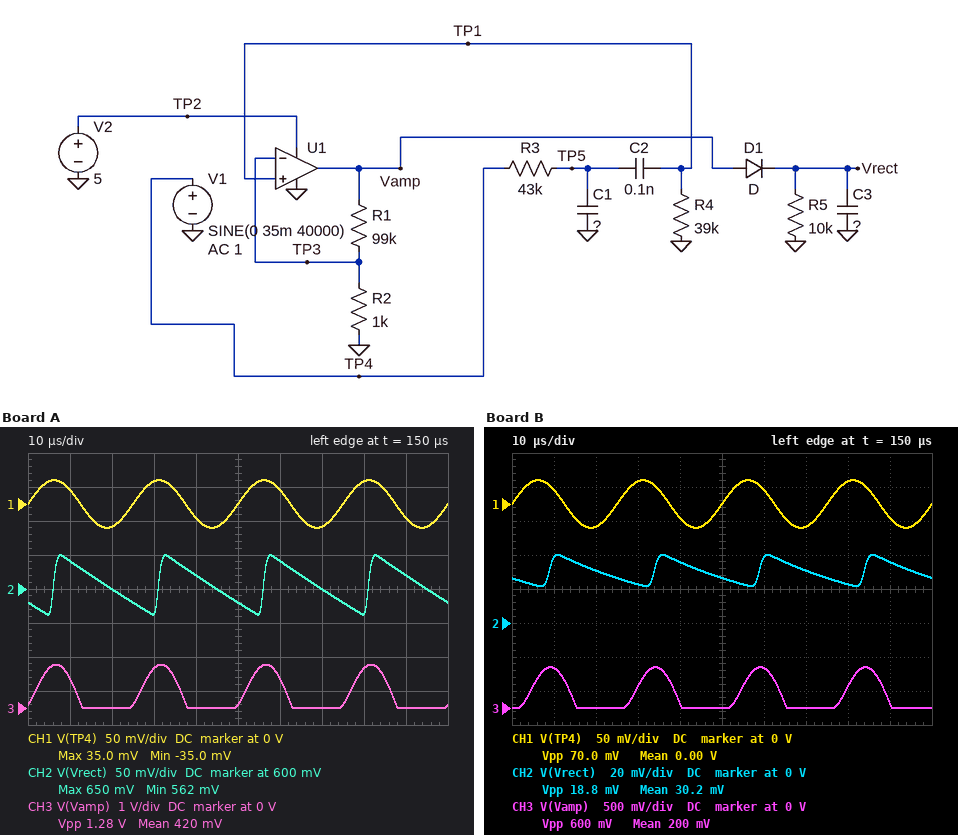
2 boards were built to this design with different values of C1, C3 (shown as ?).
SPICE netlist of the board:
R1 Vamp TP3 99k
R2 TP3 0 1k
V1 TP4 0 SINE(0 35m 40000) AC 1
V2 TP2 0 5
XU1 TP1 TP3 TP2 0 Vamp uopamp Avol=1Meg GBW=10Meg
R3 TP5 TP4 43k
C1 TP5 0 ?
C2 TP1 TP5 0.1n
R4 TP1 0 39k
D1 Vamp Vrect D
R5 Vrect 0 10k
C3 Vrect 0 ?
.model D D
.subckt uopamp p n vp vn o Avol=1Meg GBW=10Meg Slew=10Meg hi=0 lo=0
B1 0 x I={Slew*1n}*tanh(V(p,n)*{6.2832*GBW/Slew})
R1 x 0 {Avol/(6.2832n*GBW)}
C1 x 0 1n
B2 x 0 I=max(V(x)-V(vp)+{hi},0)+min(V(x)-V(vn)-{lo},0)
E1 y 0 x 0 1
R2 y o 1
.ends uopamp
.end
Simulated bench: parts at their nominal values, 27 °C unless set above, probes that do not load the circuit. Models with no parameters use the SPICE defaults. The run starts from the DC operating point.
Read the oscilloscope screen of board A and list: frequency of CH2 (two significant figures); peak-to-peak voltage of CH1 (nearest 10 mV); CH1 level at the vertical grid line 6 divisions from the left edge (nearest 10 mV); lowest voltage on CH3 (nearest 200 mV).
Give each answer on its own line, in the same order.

40 kHz
70 mV
20 mV
0 V
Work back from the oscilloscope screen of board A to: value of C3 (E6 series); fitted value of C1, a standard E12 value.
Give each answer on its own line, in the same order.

15 nF
33 pF
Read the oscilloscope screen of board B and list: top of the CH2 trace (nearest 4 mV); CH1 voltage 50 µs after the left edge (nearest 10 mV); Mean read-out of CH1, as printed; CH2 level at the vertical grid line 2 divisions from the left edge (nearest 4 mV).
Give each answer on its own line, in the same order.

40 mV
0 V
0.00 V
32 mV
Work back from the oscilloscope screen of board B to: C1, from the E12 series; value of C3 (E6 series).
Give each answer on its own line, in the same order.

270 pF
3.3 nF
